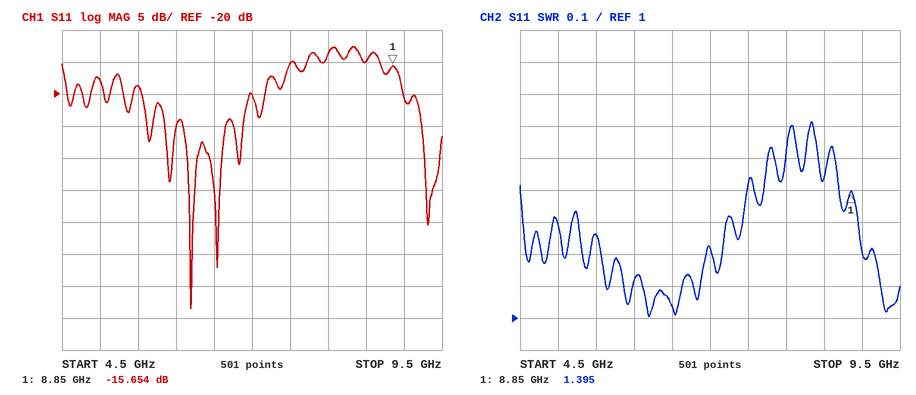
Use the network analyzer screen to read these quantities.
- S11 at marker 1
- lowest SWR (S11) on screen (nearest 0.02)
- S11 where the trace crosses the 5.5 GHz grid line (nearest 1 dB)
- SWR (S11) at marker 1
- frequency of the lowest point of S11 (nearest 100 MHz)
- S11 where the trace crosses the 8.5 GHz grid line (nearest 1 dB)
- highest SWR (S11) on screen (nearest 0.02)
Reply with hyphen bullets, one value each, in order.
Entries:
- -15.654 dB
- 1.00
- -19 dB
- 1.395
- 6.2 GHz
- -15 dB
- 1.62
